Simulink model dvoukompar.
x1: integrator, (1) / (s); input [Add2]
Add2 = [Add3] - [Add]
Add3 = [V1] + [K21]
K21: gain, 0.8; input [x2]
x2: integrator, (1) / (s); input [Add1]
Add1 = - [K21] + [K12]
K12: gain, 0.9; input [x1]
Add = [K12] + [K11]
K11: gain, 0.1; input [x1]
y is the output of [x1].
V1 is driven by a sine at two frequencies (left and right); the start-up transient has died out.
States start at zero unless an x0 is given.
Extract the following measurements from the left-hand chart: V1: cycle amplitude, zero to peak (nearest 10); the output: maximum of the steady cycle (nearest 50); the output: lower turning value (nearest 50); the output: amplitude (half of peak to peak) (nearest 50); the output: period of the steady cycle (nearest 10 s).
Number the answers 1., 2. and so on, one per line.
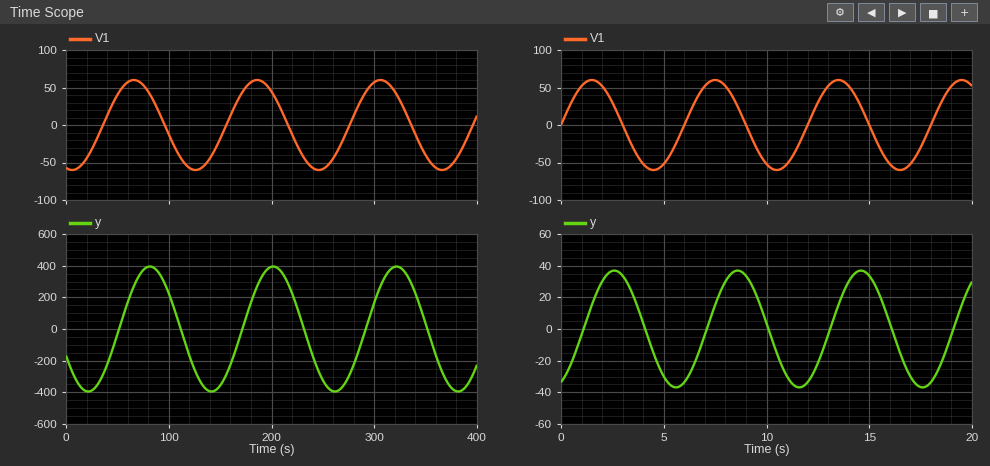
1. 60
2. 400
3. -400
4. 400
5. 120 s
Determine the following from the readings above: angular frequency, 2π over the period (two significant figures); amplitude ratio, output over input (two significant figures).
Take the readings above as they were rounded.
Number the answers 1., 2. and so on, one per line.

1. 0.052 rad/s
2. 6.7
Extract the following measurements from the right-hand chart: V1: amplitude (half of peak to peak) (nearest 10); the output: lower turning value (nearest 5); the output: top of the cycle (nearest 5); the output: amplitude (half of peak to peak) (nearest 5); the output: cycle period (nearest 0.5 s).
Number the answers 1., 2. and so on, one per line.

1. 60
2. -35
3. 35
4. 35
5. 6.0 s
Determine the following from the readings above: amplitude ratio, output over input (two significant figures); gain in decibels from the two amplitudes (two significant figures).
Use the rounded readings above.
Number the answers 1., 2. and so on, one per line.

1. 0.58
2. -4.7 dB
